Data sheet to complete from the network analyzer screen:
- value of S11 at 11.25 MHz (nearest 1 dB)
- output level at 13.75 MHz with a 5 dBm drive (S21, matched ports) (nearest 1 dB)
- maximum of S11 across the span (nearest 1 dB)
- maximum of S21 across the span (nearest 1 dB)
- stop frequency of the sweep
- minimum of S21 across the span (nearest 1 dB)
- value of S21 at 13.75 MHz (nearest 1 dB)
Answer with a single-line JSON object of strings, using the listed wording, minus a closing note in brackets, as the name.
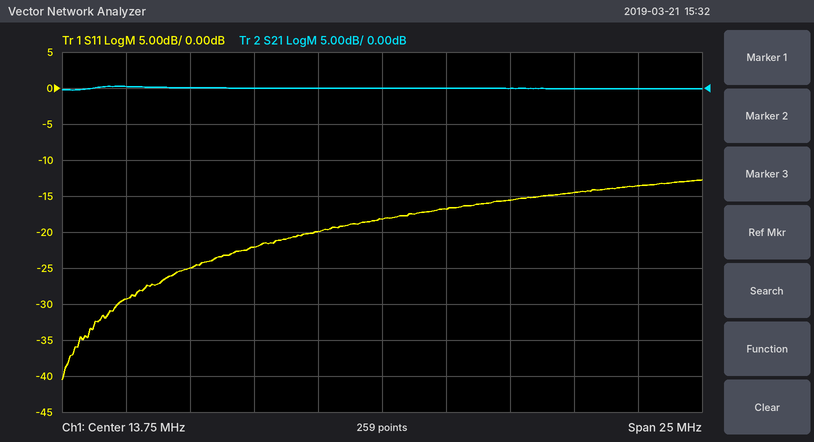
{"value of S11 at 11.25 MHz": "-20 dB", "output level at 13.75 MHz with a 5 dBm drive (S21, matched ports)": "5 dBm", "maximum of S11 across the span": "-13 dB", "maximum of S21 across the span": "0 dB", "stop frequency of the sweep": "26.25 MHz", "minimum of S21 across the span": "0 dB", "value of S21 at 13.75 MHz": "0 dB"}
